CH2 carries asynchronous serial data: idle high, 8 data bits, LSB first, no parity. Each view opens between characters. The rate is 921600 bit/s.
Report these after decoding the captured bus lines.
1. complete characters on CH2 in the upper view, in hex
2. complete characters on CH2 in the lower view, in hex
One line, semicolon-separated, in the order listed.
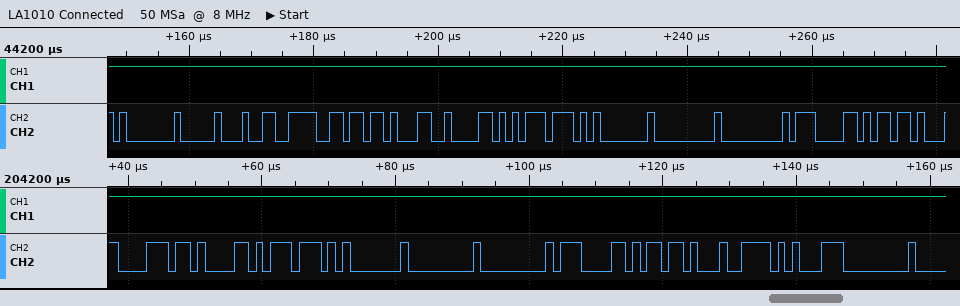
01, 10, E6, B6, 31, 58, 77, 01, 00, 00, 87, 6D; B8, 61, 77, 01, 00, 00, 87, 6D, E4, C5, 00
